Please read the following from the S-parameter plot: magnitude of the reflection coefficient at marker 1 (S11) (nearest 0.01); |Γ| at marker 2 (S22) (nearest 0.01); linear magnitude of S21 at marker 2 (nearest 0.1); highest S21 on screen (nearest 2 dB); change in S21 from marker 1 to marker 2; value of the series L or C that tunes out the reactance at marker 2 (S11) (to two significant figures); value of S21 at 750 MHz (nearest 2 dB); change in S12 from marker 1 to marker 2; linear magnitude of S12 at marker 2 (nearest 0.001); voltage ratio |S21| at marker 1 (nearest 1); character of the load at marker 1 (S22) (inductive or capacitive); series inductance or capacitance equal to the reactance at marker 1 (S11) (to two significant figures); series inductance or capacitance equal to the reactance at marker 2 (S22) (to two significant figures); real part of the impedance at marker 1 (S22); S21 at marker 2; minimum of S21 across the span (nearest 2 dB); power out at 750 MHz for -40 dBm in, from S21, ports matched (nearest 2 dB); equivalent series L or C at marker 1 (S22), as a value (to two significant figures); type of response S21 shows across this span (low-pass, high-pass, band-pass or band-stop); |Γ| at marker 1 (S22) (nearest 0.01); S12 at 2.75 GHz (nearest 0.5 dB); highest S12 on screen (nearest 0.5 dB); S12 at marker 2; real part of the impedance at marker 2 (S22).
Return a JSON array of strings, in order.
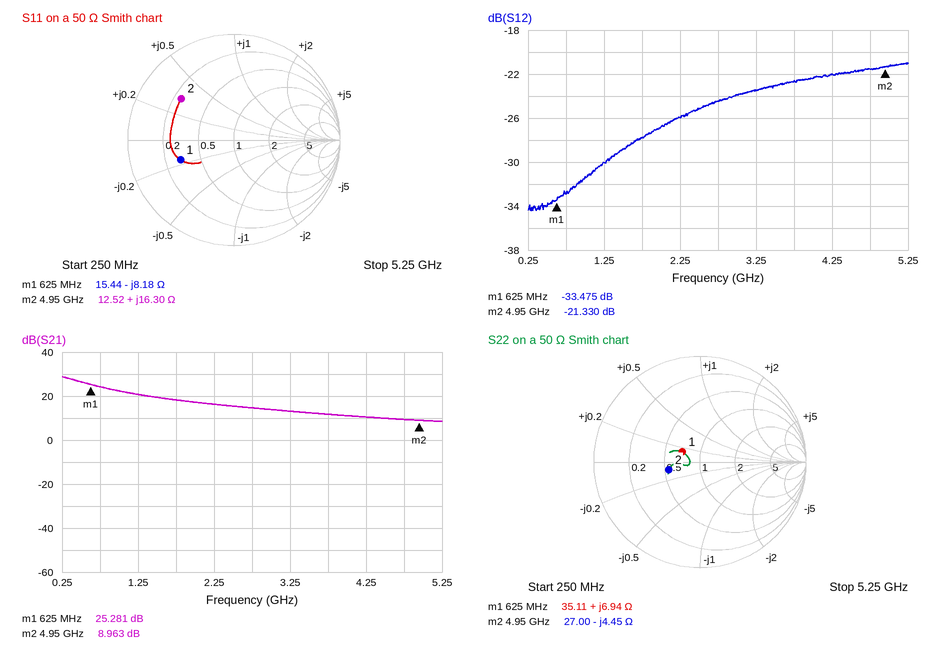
["0.54", "0.30", "2.8", "28 dB", "-16.318 dB", "2.0 pF", "24 dB", "12.145 dB", "0.086", "18", "inductive", "31 pF", "7.2 pF", "35.11 Ω", "8.963 dB", "8 dB", "-16 dBm", "1.8 nH", "low-pass", "0.19", "-24.5 dB", "-21.0 dB", "-21.330 dB", "27.00 Ω"]
